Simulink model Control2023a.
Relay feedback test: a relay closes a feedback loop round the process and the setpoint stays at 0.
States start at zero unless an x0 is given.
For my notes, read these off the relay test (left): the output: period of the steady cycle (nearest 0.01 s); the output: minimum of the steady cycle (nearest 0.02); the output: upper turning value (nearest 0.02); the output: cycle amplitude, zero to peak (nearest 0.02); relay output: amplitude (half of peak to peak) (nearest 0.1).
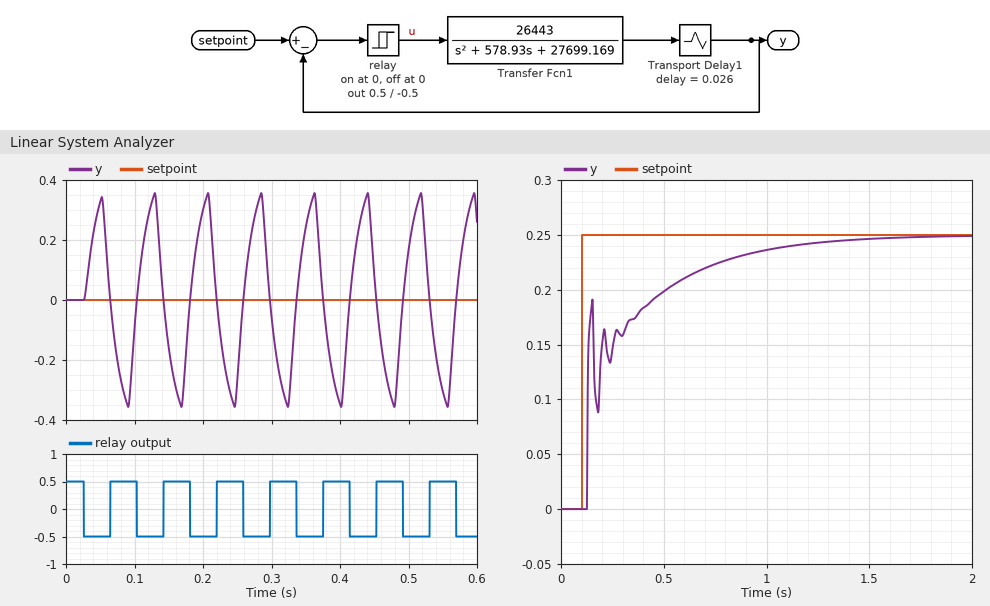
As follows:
0.08 s
-0.36
0.36
0.36
0.5
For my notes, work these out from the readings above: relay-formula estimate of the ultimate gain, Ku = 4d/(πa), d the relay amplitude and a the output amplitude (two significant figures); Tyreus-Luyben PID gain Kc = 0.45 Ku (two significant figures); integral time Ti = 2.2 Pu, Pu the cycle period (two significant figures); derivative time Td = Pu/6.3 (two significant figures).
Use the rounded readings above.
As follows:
1.8
0.81
0.18 s
0.013 s
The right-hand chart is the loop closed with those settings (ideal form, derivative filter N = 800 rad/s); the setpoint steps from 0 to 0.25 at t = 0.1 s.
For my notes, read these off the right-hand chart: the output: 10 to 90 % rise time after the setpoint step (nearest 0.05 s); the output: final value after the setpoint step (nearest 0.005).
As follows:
0.65 s
0.250
